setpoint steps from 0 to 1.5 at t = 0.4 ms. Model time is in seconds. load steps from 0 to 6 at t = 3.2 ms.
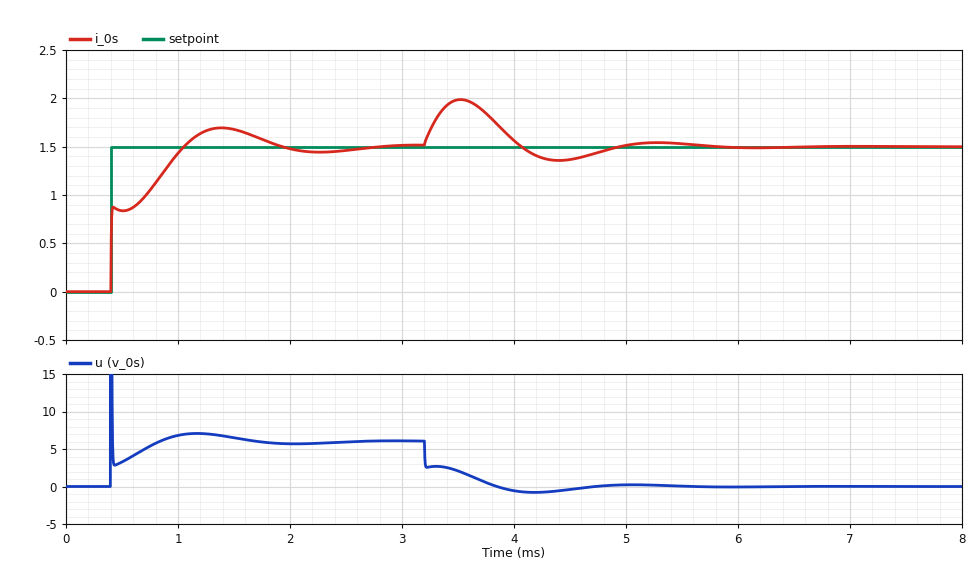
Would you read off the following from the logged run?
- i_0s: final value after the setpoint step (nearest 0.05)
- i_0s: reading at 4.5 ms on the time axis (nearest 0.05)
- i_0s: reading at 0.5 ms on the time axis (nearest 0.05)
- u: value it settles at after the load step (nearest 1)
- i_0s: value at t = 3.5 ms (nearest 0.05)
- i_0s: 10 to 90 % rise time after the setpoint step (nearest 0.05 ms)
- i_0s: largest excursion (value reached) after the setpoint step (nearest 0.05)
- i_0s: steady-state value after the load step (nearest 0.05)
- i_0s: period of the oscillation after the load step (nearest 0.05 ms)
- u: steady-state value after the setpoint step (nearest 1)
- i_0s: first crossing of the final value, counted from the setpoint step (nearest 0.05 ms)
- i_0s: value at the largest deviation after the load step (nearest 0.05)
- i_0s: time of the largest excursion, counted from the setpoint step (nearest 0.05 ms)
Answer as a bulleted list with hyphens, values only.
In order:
- 1.50
- 1.35
- 0.85
- 0
- 2.00
- 0.55 ms
- 1.70
- 1.50
- 1.75 ms
- 6
- 0.65 ms
- 2.00
- 1.00 ms
